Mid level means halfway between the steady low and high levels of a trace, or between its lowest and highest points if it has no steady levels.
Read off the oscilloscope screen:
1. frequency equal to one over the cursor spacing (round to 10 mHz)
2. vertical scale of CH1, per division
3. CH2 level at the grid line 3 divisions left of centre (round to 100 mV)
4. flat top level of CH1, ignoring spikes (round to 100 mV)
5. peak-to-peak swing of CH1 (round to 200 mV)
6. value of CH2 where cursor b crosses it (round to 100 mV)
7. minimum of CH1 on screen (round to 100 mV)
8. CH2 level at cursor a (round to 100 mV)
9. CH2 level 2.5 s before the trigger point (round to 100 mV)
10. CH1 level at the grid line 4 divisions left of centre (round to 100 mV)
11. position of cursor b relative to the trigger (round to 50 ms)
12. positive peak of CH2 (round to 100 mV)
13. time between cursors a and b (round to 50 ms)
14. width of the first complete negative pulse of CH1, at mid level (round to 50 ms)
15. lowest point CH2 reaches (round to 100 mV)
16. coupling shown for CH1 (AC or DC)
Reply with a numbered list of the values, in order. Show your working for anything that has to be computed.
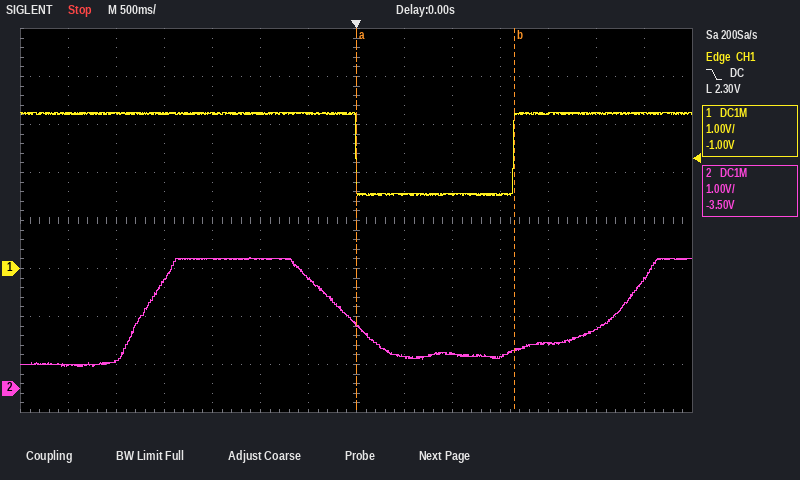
1. 1 / 1.65 s ≈ 610 mHz
2. 1 V
3. 2.7 V
4. 3.2 V
5. 1.8 V
6. 800 mV
7. 1.5 V
8. 1.3 V
9. 600 mV
10. 3.2 V
11. +1.65 s
12. 2.7 V
13. 1.65 s
14. 1.65 s
15. 500 mV
16. DC
